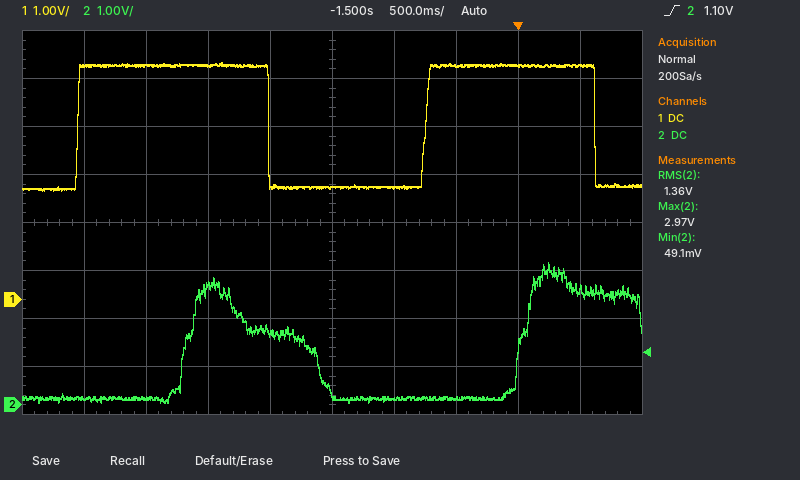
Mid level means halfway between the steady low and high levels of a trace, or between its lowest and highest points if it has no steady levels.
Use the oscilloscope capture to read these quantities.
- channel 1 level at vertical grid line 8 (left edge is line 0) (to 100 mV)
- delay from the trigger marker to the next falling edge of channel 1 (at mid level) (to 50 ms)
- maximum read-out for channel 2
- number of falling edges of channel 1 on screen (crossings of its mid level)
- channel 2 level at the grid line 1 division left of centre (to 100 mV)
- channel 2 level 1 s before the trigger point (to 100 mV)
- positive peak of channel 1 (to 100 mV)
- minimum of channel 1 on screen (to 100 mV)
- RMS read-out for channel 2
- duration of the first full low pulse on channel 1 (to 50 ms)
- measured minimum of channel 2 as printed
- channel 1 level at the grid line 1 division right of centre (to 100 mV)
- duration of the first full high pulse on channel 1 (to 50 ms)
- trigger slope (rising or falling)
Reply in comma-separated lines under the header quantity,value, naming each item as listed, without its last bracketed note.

quantity,value
channel 1 level at vertical grid line 8 (left edge is line 0),4.9 V
delay from the trigger marker to the next falling edge of channel 1 (at mid level),600 ms
maximum read-out for channel 2,2.97 V
number of falling edges of channel 1 on screen,2
channel 2 level at the grid line 1 division left of centre,1.5 V
channel 2 level 1 s before the trigger point,100 mV
positive peak of channel 1,4.9 V
minimum of channel 1 on screen,2.3 V
RMS read-out for channel 2,1.36 V
duration of the first full low pulse on channel 1,1.25 s
measured minimum of channel 2 as printed,49.1 mV
channel 1 level at the grid line 1 division right of centre,2.3 V
duration of the first full high pulse on channel 1,1.55 s
trigger slope,rising
